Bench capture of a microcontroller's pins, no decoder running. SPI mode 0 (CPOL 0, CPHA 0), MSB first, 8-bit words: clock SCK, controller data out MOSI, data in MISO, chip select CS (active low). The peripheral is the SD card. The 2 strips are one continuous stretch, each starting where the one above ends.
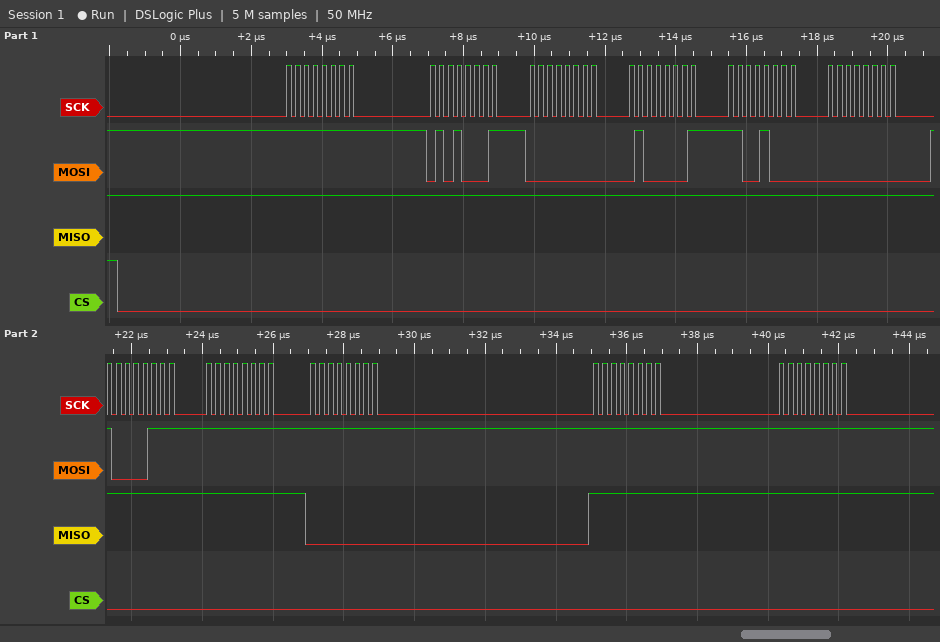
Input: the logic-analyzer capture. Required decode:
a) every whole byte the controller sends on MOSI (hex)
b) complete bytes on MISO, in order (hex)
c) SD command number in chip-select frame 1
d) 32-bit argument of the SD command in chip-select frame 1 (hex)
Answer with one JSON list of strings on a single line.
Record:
["FF 51 00 41 C8 00 87 FF FF FF FF", "FF FF FF FF FF FF FF FF 00 FF FF", "CMD17", "0x0041C800"]
